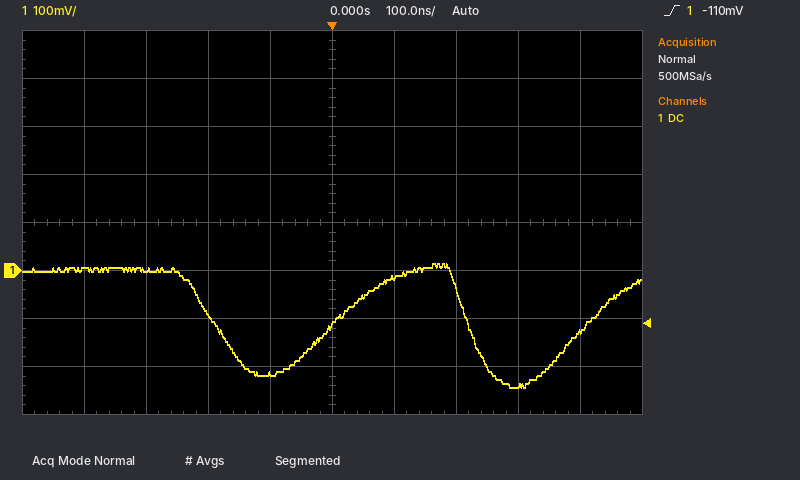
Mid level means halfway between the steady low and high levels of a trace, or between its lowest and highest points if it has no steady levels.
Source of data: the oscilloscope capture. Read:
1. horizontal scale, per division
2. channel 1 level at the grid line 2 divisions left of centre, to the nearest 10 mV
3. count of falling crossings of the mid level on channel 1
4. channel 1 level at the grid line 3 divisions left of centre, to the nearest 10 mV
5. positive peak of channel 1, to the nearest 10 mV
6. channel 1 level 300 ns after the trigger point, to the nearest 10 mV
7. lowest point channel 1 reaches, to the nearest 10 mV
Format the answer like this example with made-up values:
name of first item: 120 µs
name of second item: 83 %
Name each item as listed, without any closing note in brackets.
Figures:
horizontal scale, per division: 100 ns
channel 1 level at the grid line 2 divisions left of centre, to the nearest 10 mV: -90 mV
count of falling crossings of the mid level on channel 1: 2
channel 1 level at the grid line 3 divisions left of centre, to the nearest 10 mV: 0 mV
positive peak of channel 1, to the nearest 10 mV: 10 mV
channel 1 level 300 ns after the trigger point, to the nearest 10 mV: -240 mV
lowest point channel 1 reaches, to the nearest 10 mV: -240 mV
